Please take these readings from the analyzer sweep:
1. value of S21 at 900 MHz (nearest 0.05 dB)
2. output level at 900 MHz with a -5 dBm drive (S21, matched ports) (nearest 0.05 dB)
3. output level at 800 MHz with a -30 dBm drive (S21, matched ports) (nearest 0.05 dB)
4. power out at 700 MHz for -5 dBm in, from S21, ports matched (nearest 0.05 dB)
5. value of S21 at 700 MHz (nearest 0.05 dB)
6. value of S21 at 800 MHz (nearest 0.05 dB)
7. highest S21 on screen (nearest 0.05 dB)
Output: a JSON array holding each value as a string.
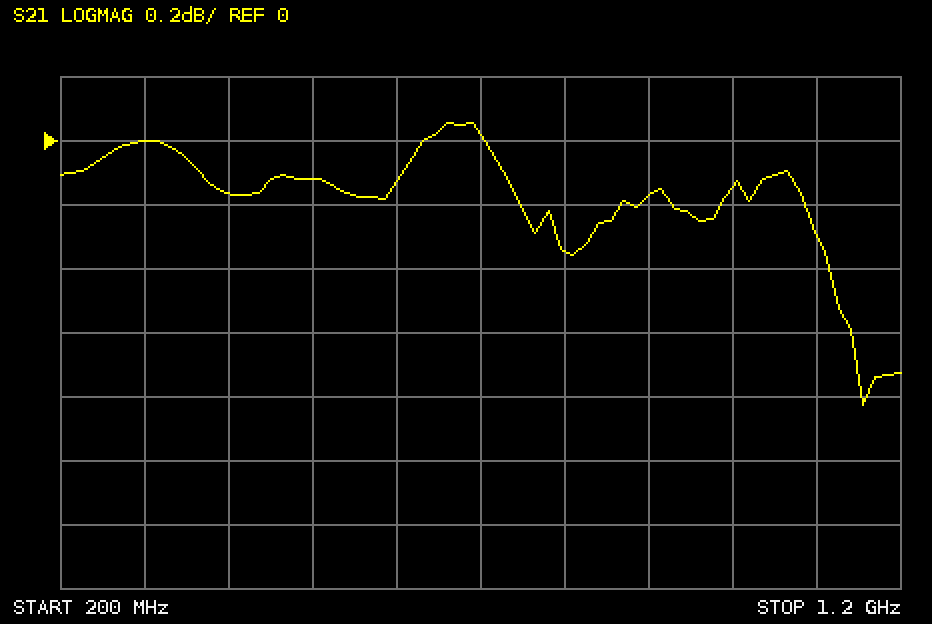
["-0.15 dB", "-5.15 dBm", "-30.35 dBm", "-5.00 dBm", "0.00 dB", "-0.35 dB", "0.05 dB"]
